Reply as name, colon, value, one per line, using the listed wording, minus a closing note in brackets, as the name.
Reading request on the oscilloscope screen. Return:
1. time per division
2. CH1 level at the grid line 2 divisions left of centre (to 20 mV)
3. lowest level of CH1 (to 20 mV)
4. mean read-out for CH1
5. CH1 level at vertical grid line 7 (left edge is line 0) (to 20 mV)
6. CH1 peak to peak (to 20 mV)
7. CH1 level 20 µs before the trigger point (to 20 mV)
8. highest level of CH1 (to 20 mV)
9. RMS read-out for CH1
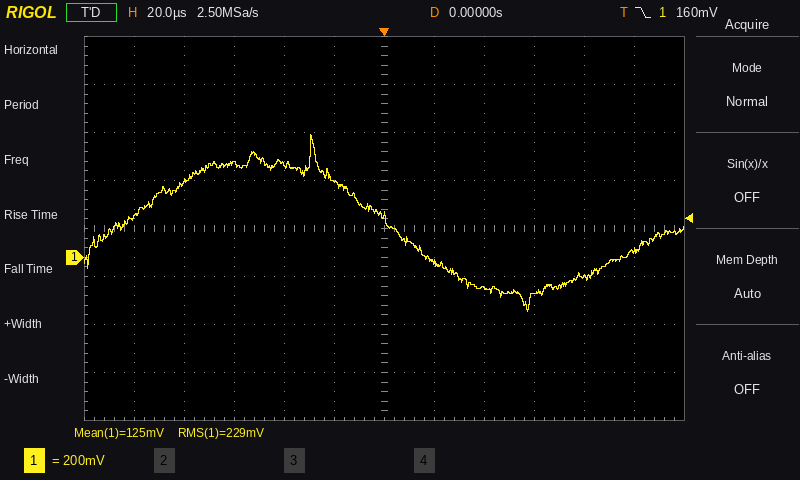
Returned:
time per division: 20 µs
CH1 level at the grid line 2 divisions left of centre: 380 mV
lowest level of CH1: -220 mV
mean read-out for CH1: 125 mV
CH1 level at vertical grid line 7 (left edge is line 0): -20 mV
CH1 peak to peak: 740 mV
CH1 level 20 µs before the trigger point: 320 mV
highest level of CH1: 520 mV
RMS read-out for CH1: 229 mV
